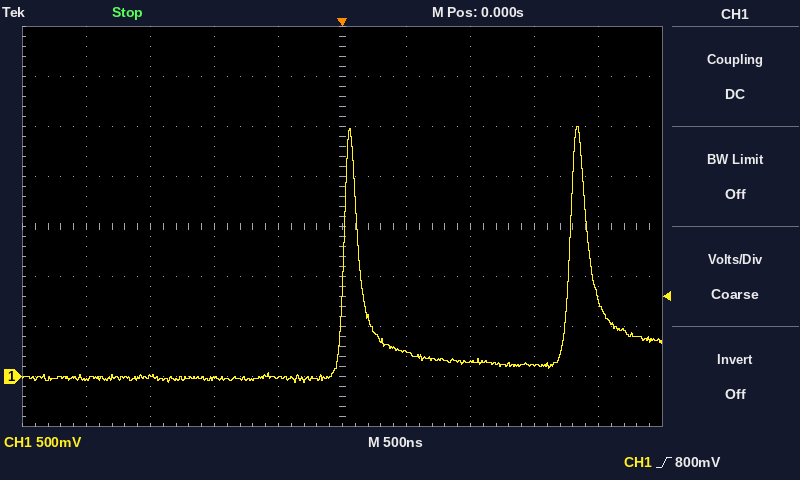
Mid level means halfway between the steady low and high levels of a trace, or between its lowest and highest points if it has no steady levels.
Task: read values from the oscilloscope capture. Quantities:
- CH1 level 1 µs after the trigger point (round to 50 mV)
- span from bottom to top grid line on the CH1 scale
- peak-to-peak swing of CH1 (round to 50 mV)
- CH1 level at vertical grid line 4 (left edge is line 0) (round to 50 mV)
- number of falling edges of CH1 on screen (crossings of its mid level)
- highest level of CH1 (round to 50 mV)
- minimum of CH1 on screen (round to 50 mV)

150 mV
4 V
2.55 V
0 mV
2
2.50 V
-50 mV
